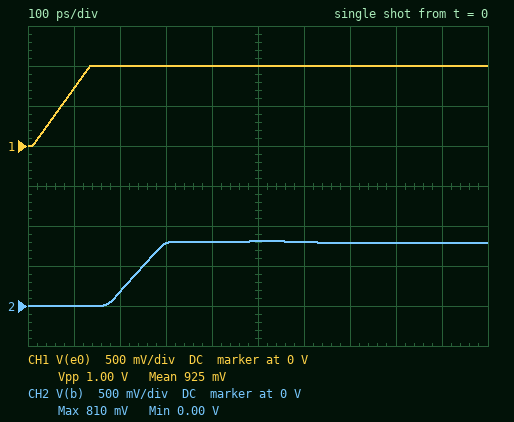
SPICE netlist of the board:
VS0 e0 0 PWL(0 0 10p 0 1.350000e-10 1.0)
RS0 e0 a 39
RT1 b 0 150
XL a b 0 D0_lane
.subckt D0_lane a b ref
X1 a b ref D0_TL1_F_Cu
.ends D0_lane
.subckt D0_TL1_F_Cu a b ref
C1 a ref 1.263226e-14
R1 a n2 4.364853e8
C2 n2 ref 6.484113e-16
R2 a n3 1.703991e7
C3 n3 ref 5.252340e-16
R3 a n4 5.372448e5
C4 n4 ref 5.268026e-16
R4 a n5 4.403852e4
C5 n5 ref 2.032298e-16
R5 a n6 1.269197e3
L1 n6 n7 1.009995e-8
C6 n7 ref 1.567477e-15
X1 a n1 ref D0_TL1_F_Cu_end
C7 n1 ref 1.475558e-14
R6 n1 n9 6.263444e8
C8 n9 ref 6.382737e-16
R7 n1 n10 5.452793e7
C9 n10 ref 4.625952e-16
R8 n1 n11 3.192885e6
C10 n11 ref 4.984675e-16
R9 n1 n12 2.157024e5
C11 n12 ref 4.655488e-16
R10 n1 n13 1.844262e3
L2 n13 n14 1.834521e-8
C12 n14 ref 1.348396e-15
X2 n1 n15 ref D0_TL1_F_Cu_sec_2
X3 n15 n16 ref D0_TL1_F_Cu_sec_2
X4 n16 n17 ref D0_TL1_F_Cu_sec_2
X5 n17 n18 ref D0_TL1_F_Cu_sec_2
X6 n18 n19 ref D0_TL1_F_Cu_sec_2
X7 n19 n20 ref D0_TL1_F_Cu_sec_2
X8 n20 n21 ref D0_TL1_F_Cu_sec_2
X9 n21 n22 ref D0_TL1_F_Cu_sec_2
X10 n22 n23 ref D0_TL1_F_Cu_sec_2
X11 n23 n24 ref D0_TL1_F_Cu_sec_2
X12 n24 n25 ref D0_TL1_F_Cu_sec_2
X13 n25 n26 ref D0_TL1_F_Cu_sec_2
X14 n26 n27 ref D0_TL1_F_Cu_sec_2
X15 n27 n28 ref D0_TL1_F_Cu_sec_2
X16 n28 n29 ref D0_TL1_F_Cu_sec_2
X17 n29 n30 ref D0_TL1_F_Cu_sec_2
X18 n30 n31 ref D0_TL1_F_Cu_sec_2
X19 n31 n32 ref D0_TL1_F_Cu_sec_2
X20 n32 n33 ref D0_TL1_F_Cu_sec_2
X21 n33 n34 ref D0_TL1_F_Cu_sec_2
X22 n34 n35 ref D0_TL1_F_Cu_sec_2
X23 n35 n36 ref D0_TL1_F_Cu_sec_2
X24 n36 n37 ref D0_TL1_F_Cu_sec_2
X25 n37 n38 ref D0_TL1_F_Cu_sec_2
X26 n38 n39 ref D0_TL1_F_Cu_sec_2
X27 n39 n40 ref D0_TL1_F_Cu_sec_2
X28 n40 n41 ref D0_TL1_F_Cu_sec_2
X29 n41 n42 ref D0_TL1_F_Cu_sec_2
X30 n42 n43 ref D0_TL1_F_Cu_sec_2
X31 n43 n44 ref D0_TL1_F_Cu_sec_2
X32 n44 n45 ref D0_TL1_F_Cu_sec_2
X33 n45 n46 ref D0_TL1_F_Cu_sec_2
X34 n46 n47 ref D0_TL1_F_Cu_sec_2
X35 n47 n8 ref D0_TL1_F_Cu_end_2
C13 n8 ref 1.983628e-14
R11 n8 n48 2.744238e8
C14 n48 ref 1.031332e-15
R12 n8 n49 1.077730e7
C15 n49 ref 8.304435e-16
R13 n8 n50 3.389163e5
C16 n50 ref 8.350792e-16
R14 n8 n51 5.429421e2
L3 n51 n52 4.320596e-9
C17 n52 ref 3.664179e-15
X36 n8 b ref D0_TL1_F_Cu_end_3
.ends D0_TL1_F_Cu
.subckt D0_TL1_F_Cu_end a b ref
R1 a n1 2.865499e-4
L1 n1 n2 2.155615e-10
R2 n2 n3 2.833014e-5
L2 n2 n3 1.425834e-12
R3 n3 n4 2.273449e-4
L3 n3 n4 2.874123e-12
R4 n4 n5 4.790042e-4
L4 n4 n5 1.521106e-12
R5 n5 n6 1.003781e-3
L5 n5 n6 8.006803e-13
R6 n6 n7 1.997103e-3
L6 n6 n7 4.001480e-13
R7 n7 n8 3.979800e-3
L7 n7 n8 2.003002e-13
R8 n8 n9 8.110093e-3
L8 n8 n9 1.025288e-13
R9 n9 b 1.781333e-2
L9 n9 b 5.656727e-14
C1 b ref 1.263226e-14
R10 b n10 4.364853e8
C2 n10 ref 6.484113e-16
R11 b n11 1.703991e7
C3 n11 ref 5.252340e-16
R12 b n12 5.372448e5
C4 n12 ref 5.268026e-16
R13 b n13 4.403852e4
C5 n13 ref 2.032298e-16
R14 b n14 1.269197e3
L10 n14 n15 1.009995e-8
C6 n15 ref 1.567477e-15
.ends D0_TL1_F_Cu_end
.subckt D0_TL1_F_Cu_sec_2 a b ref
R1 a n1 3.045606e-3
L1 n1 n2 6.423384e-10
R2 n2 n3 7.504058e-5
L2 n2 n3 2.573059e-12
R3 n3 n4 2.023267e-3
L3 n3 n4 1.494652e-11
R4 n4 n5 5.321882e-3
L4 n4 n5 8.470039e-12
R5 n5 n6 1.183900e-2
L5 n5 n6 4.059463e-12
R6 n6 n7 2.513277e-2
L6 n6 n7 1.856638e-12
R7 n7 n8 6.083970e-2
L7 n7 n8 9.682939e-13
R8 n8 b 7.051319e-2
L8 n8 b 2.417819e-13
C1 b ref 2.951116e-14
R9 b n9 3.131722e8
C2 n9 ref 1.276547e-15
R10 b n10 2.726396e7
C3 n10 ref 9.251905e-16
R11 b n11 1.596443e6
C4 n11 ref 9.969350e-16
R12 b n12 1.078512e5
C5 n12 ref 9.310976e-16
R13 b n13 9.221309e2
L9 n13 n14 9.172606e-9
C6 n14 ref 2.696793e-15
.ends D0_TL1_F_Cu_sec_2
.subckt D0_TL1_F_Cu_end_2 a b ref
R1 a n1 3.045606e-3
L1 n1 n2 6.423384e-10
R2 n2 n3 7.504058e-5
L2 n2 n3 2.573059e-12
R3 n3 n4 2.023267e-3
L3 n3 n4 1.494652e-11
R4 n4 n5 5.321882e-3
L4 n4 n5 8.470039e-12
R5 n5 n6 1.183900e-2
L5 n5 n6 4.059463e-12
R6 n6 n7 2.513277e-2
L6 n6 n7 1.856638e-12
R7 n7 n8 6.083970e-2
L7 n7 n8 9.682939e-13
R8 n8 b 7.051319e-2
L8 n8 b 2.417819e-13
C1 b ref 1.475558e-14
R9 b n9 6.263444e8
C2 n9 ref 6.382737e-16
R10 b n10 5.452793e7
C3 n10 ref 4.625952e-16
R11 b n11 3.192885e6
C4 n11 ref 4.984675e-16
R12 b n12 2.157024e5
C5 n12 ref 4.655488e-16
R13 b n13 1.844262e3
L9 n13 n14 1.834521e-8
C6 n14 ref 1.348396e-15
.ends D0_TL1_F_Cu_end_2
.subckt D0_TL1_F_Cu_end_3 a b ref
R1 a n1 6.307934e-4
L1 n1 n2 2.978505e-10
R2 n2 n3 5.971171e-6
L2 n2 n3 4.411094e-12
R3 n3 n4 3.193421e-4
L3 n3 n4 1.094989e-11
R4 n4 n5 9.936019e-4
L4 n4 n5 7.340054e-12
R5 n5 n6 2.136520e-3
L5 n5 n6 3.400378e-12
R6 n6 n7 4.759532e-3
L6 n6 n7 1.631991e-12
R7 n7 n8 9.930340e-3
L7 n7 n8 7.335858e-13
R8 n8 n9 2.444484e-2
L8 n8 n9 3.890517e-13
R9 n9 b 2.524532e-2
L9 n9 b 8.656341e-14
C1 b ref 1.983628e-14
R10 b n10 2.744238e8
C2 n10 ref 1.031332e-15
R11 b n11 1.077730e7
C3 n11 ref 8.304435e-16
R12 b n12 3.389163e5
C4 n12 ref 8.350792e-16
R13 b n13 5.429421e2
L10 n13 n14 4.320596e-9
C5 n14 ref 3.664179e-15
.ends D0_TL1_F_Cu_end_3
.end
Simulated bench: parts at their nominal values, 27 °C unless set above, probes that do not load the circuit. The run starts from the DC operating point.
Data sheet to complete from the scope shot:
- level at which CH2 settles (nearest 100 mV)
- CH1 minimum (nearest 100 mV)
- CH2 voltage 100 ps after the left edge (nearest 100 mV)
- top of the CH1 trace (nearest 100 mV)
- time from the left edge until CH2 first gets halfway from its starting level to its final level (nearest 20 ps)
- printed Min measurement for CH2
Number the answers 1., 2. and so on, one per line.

1. 800 mV
2. 0 V
3. 0 V
4. 1.0 V
5. 240 ps
6. 0.00 V
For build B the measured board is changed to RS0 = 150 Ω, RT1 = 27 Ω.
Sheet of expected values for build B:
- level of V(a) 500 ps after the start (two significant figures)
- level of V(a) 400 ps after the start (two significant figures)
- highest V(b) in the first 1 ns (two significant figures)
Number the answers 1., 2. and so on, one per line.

1. 150 mV
2. 300 mV
3. 160 mV
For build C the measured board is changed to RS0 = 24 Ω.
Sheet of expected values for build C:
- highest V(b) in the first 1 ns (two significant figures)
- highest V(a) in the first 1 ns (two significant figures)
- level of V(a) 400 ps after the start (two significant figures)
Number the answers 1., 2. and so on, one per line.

1. 890 mV
2. 860 mV
3. 850 mV
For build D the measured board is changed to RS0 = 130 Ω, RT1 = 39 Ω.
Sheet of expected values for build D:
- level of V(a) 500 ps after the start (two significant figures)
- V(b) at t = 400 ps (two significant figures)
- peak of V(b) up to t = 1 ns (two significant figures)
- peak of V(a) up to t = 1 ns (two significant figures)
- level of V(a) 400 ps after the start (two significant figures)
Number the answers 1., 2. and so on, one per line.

1. 240 mV
2. 220 mV
3. 230 mV
4. 520 mV
5. 360 mV
